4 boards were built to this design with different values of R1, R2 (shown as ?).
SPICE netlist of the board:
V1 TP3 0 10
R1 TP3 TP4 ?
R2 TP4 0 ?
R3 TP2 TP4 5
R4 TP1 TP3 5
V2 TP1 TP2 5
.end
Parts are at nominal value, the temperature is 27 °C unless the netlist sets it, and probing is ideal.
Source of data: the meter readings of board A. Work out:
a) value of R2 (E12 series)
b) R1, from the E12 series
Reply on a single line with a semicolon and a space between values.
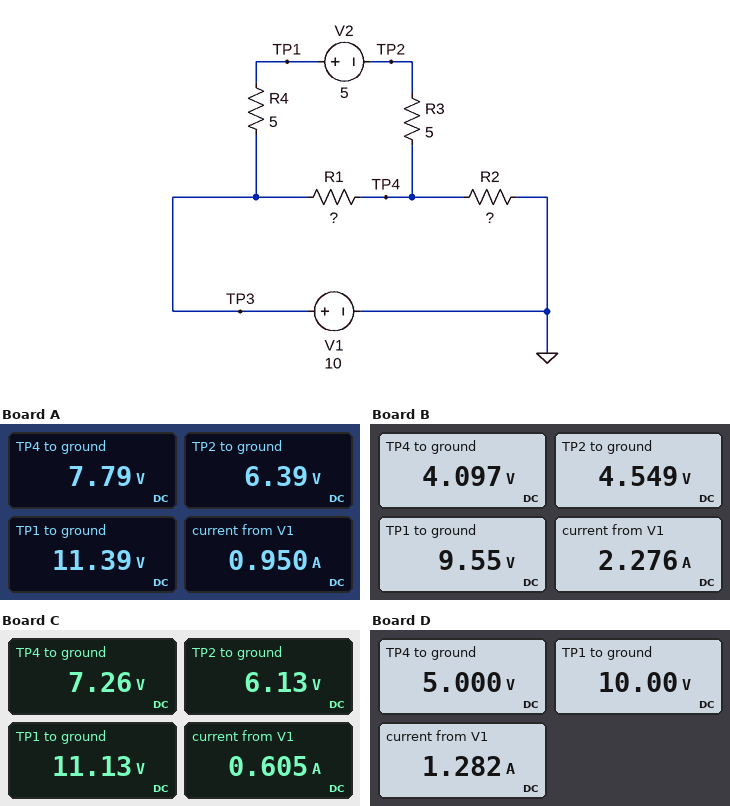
8.2 Ω; 1.8 Ω
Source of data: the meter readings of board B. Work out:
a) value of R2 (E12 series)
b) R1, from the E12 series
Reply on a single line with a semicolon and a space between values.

1.8 Ω; 2.7 Ω
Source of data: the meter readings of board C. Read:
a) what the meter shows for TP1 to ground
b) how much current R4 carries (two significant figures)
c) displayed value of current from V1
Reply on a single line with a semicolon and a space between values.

11.13 V; 230 mA; 0.605 A
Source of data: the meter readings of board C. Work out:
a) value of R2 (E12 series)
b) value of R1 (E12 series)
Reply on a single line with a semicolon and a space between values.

12 Ω; 3.3 Ω
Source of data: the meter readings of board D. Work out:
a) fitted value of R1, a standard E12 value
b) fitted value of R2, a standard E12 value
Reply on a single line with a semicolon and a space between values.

3.9 Ω; 3.9 Ω
